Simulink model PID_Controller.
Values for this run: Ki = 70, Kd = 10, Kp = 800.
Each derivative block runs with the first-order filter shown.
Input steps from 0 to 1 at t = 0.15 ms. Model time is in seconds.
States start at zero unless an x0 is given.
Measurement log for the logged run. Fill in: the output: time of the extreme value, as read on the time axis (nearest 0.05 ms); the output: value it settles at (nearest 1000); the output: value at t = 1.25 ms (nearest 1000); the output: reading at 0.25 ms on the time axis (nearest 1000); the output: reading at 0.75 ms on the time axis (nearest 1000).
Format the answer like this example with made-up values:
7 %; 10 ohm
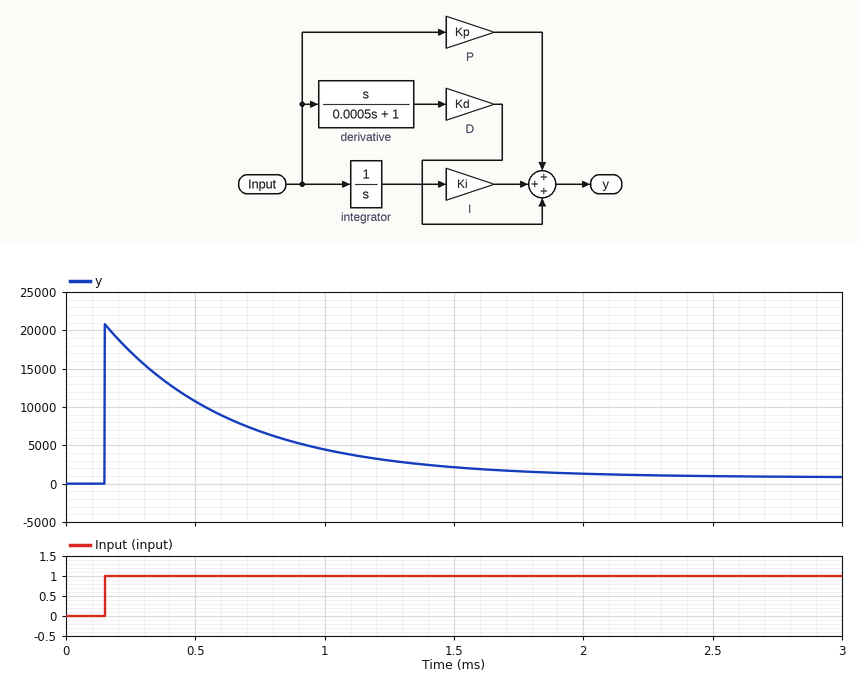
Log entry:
0.15 ms; 1000; 3000; 17000; 7000
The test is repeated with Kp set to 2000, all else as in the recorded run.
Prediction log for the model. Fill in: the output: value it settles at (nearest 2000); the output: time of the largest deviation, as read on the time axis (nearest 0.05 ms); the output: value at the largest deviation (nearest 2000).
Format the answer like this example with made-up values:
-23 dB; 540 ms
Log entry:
2000; 0.15 ms; 22000
